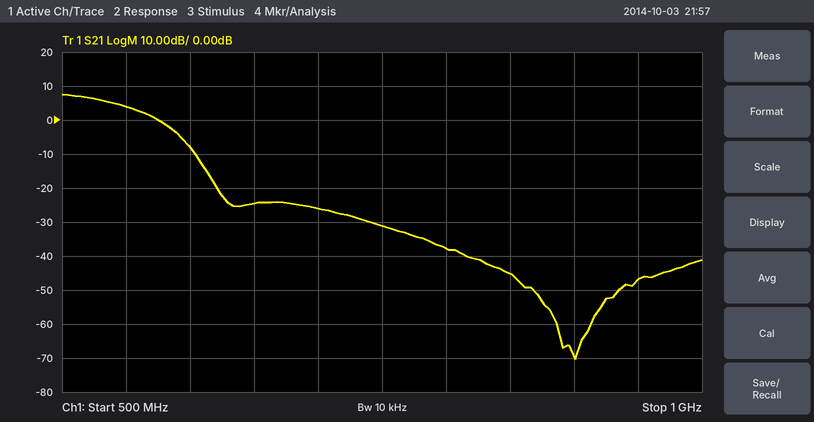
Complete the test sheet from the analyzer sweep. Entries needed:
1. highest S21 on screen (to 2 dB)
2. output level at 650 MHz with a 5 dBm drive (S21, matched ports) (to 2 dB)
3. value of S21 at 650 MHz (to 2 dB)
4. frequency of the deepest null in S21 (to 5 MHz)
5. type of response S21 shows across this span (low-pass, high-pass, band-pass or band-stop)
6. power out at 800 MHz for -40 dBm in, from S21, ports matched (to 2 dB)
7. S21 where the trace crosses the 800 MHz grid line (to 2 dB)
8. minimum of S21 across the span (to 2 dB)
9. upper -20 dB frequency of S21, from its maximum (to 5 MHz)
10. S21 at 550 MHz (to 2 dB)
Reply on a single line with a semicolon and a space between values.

8 dB; -20 dBm; -24 dB; 900 MHz; low-pass; -78 dBm; -38 dB; -70 dB; 610 MHz; 4 dB
